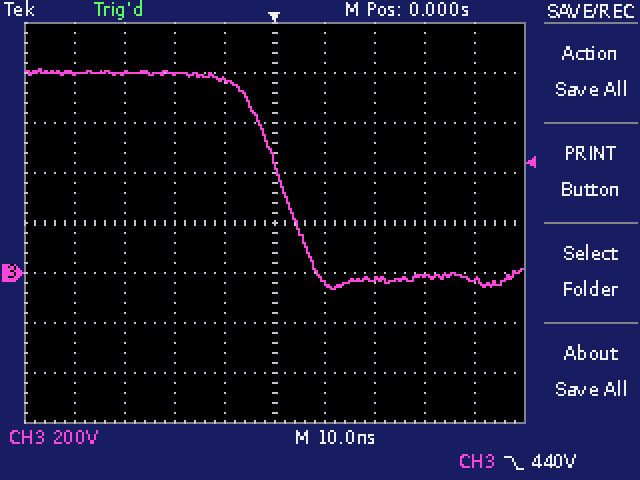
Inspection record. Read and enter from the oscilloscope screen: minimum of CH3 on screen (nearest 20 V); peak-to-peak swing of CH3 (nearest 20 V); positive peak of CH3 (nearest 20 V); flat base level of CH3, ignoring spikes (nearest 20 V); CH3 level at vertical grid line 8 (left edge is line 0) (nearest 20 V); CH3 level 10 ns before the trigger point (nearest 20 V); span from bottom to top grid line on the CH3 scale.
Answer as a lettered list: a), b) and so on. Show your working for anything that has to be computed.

a) -60 V
b) 820 V − (-60 V) = 880 V
c) 820 V
d) -20 V
e) -20 V
f) 780 V
g) 1.6 kV
